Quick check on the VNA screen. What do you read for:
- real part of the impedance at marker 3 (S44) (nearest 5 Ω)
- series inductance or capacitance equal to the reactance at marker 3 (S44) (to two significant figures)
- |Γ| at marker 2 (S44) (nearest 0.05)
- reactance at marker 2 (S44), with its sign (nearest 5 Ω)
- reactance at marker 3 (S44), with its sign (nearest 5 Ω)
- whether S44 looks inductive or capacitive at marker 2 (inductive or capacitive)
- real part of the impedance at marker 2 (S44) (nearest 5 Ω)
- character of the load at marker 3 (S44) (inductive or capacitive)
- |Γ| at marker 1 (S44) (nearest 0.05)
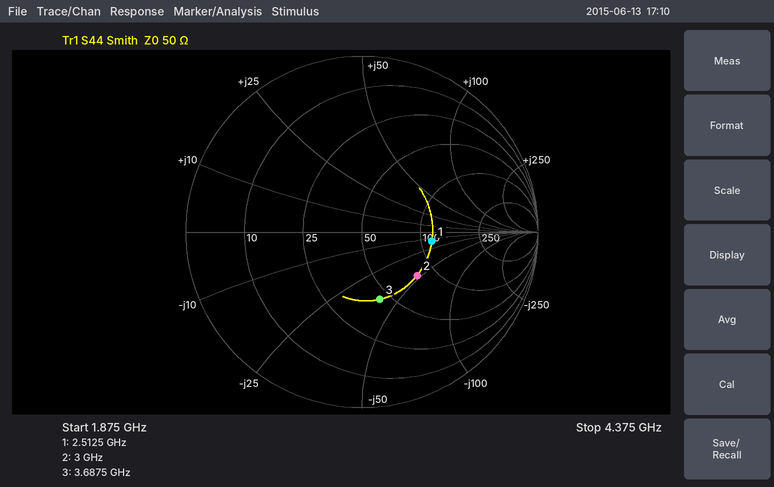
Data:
45 Ω
1.1 pF
0.40
-45 Ω
-40 Ω
capacitive
80 Ω
capacitive
0.40
